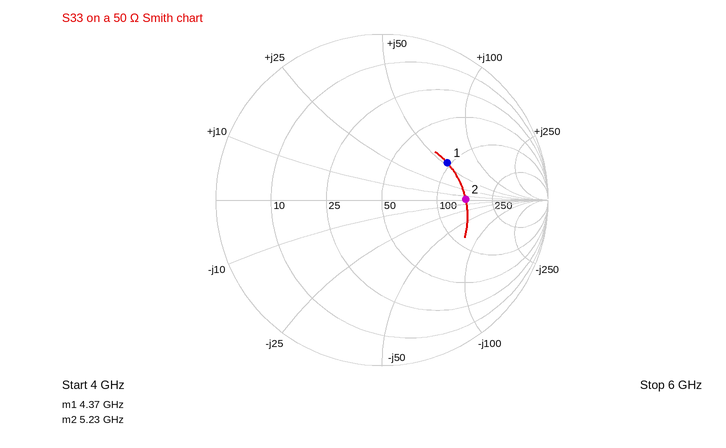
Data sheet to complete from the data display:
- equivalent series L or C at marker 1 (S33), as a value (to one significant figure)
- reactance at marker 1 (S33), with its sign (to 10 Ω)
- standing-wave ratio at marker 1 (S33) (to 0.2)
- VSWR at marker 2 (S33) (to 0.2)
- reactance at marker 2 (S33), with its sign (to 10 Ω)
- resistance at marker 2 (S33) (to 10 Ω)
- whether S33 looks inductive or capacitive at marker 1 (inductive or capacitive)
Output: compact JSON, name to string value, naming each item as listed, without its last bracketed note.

{"equivalent series L or C at marker 1 (S33), as a value": "2 nH", "reactance at marker 1 (S33), with its sign": "+50 Ω", "standing-wave ratio at marker 1 (S33)": "2.6", "VSWR at marker 2 (S33)": "3.0", "reactance at marker 2 (S33), with its sign": "0 Ω", "resistance at marker 2 (S33)": "150 Ω", "whether S33 looks inductive or capacitive at marker 1": "inductive"}
